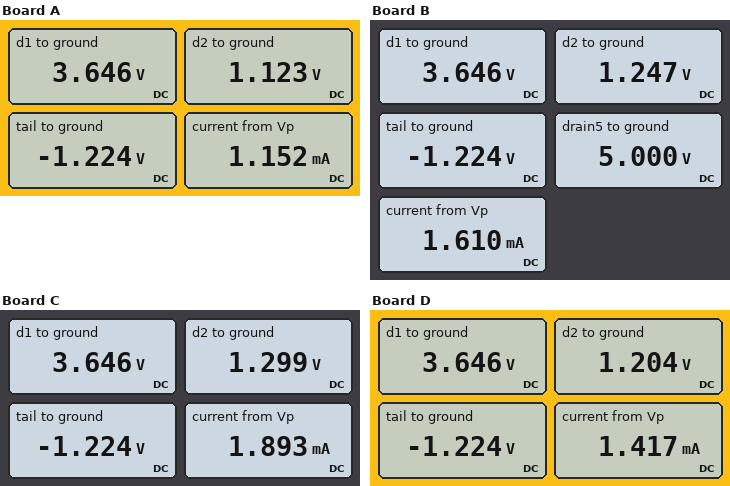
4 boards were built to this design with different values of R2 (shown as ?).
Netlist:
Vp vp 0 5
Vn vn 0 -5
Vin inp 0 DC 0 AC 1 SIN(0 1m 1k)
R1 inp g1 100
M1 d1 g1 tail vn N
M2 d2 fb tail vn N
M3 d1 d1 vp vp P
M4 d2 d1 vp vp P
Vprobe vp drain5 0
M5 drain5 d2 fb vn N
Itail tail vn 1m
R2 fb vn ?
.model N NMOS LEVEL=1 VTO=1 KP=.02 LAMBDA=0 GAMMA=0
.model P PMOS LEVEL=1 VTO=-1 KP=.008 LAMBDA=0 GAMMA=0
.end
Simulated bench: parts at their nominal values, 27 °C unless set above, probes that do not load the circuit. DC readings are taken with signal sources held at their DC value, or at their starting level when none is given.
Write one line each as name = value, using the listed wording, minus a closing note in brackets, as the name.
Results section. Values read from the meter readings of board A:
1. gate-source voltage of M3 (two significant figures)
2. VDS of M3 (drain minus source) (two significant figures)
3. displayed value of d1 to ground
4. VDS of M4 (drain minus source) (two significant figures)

gate-source voltage of M3 = -1.4 V
VDS of M3 (drain minus source) = -1.4 V
displayed value of d1 to ground = 3.646 V
VDS of M4 (drain minus source) = -3.9 V
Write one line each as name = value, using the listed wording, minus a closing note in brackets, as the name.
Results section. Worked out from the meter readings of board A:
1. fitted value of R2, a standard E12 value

fitted value of R2, a standard E12 value = 33 kΩ
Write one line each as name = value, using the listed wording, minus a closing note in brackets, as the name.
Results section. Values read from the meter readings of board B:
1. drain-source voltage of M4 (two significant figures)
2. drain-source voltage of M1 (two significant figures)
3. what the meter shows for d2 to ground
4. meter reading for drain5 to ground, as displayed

drain-source voltage of M4 = -3.8 V
drain-source voltage of M1 = 4.9 V
what the meter shows for d2 to ground = 1.247 V
meter reading for drain5 to ground, as displayed = 5.000 V
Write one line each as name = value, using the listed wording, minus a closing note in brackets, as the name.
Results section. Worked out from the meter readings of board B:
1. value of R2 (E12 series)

value of R2 = 8.2 kΩ
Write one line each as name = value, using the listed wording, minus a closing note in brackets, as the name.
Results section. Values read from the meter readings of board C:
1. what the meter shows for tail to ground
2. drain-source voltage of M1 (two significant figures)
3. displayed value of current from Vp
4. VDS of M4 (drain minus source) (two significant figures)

what the meter shows for tail to ground = -1.224 V
drain-source voltage of M1 = 4.9 V
displayed value of current from Vp = 1.893 mA
VDS of M4 (drain minus source) = -3.7 V
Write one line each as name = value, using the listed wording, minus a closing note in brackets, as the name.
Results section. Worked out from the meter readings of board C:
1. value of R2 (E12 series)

value of R2 = 5.6 kΩ
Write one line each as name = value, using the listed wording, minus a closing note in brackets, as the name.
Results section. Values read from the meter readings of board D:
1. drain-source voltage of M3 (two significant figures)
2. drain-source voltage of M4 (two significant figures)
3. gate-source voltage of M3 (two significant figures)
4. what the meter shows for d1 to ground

drain-source voltage of M3 = -1.4 V
drain-source voltage of M4 = -3.8 V
gate-source voltage of M3 = -1.4 V
what the meter shows for d1 to ground = 3.646 V
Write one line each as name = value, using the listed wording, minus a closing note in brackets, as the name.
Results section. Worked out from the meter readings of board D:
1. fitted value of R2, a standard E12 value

fitted value of R2, a standard E12 value = 12 kΩ
